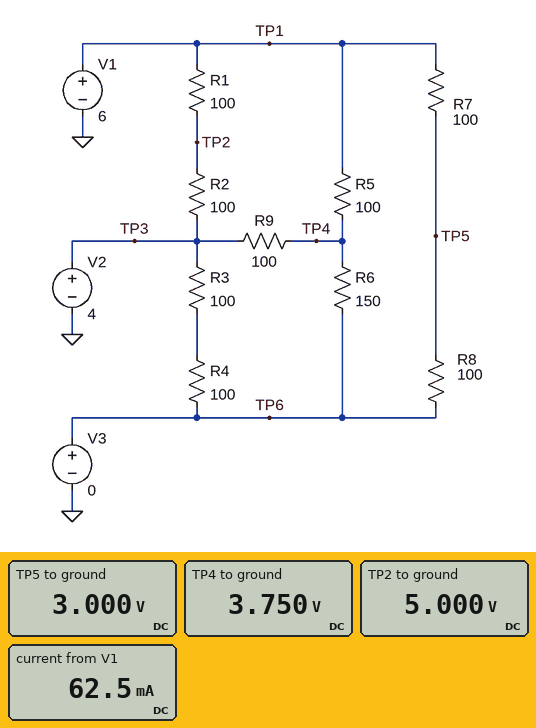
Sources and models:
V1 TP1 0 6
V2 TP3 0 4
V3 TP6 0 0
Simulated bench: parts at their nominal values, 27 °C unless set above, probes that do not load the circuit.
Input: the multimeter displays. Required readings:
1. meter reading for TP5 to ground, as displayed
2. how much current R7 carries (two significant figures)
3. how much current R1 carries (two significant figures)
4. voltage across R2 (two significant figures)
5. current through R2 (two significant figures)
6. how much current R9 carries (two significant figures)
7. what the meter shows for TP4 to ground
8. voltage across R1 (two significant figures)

3.000 V
30 mA
10 mA
1.0 V
10 mA
2.5 mA
3.750 V
1.0 V
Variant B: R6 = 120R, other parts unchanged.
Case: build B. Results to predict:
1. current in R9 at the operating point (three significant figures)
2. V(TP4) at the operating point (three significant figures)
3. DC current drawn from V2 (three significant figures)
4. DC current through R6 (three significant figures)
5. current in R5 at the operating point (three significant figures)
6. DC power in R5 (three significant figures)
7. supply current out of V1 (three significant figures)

4.71 mA
3.53 V
14.7 mA
29.4 mA
24.7 mA
61.0 mW
64.7 mA
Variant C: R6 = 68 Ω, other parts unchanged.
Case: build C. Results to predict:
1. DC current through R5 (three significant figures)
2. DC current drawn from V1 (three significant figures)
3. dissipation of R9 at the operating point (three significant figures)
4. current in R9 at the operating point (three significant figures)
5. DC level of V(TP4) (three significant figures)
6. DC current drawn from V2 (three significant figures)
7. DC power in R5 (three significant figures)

31.2 mA
71.2 mA
12.5 mW
11.2 mA
2.88 V
21.2 mA
97.3 mW
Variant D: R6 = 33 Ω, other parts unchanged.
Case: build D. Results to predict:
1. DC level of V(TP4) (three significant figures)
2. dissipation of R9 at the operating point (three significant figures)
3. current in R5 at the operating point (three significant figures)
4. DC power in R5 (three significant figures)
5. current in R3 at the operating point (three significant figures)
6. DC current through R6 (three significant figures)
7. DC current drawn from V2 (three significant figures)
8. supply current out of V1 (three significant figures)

1.99 V
40.5 mW
40.1 mA
161 mW
20.0 mA
60.2 mA
30.1 mA
80.1 mA
